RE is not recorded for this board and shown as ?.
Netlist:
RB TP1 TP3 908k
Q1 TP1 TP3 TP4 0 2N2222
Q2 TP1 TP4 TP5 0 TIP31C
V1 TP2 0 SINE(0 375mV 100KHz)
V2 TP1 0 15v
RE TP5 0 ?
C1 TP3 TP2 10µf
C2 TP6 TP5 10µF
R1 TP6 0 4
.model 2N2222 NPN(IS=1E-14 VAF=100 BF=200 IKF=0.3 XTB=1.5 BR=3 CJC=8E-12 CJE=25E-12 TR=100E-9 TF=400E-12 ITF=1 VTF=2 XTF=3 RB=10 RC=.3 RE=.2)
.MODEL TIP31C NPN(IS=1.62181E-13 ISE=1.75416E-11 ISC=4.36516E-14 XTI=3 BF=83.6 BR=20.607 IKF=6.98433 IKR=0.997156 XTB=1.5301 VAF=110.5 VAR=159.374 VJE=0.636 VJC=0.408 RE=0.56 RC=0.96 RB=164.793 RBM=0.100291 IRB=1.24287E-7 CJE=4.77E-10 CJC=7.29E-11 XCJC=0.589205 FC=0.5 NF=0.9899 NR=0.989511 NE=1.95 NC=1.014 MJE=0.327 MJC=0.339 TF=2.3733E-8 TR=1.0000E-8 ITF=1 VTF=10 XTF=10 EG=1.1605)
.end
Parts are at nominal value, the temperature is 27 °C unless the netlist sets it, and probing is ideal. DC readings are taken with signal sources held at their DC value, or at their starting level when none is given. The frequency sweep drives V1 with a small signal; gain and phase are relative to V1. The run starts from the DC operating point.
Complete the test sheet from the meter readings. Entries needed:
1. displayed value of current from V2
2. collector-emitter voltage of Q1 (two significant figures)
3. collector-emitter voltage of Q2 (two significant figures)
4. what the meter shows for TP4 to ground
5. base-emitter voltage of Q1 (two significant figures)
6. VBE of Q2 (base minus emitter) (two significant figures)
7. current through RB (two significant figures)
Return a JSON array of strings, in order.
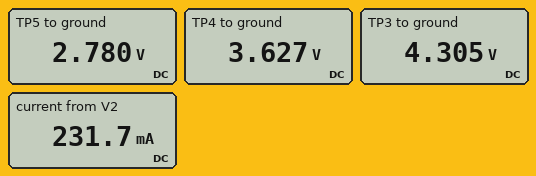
["231.7 mA", "11 V", "12 V", "3.627 V", "680 mV", "850 mV", "12 µA"]
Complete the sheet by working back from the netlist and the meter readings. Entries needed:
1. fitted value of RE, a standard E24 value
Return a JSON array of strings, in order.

["12 Ω"]
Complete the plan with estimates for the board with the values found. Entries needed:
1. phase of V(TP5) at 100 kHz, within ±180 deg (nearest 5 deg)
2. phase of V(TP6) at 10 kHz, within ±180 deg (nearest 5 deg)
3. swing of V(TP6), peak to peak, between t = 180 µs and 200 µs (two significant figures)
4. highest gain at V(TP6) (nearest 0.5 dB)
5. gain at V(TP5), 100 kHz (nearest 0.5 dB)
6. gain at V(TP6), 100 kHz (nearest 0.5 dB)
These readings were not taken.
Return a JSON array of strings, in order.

["-5 deg", "20 deg", "590 mV", "-2.0 dB", "-2.0 dB", "-2.0 dB"]
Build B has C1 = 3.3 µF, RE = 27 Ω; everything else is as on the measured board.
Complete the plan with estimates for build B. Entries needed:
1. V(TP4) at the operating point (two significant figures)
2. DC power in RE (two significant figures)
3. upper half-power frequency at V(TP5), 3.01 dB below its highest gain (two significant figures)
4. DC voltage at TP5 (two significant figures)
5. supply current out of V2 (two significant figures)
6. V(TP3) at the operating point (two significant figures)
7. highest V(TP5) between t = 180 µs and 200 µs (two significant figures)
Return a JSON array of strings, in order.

["5.7 V", "890 mW", "780 kHz", "4.9 V", "180 mA", "6.4 V", "5.2 V"]
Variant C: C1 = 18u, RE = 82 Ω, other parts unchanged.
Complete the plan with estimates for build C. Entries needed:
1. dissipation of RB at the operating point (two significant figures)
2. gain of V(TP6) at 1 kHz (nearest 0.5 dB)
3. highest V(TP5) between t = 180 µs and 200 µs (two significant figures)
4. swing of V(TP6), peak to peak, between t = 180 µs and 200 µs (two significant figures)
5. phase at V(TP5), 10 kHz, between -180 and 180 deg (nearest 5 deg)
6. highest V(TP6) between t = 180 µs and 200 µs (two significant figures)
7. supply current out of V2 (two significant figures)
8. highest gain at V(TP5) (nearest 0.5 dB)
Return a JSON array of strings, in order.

["29 µW", "-12.5 dB", "8.7 V", "550 mV", "-5 deg", "280 mV", "100 mA", "0 dB"]
